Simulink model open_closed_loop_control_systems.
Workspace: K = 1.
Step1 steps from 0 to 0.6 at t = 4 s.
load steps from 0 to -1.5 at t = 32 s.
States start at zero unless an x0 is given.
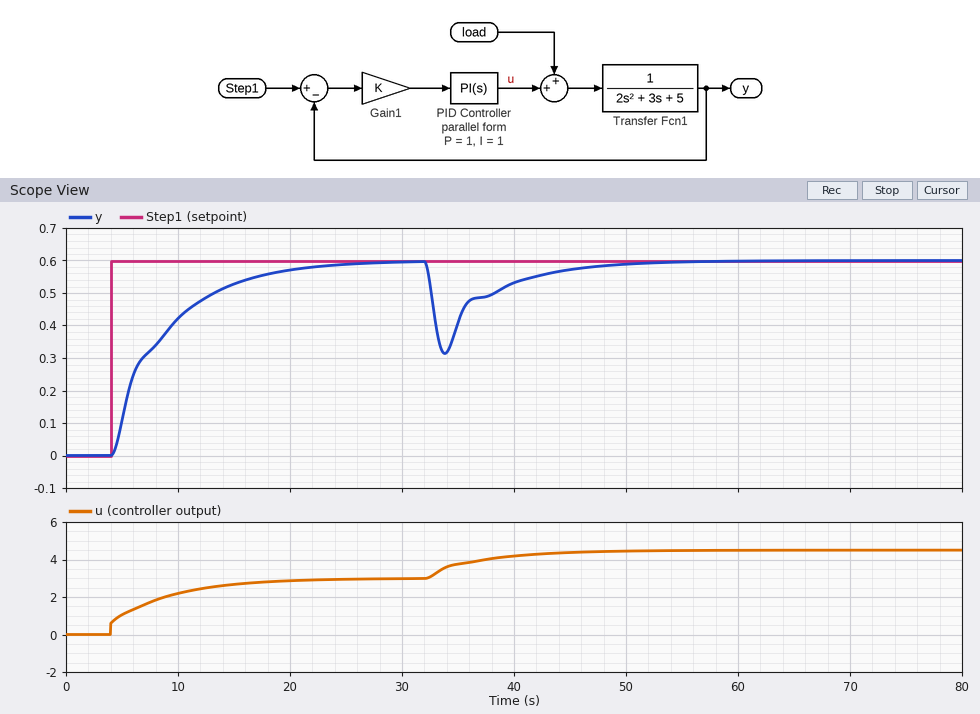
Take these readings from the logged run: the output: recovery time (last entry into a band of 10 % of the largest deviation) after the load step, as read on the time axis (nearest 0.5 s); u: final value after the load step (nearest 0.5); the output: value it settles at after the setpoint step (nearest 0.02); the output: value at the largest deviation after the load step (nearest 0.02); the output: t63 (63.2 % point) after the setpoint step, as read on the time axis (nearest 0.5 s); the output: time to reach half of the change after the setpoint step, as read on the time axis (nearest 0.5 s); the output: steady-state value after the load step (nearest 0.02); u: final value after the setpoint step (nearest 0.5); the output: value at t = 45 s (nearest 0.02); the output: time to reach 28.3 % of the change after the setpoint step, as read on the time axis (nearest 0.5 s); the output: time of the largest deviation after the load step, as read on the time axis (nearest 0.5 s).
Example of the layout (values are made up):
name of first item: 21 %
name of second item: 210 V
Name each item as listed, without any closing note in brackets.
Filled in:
the output: recovery time (last entry into a band of 10 % of the largest deviation) after the load step, as read on the time axis: 45.0 s
u: final value after the load step: 4.5
the output: value it settles at after the setpoint step: 0.60
the output: value at the largest deviation after the load step: 0.32
the output: t63 (63.2 % point) after the setpoint step, as read on the time axis: 9.0 s
the output: time to reach half of the change after the setpoint step, as read on the time axis: 7.0 s
the output: steady-state value after the load step: 0.60
u: final value after the setpoint step: 3.0
the output: value at t = 45 s: 0.58
the output: time to reach 28.3 % of the change after the setpoint step, as read on the time axis: 5.5 s
the output: time of the largest deviation after the load step, as read on the time axis: 34.0 s
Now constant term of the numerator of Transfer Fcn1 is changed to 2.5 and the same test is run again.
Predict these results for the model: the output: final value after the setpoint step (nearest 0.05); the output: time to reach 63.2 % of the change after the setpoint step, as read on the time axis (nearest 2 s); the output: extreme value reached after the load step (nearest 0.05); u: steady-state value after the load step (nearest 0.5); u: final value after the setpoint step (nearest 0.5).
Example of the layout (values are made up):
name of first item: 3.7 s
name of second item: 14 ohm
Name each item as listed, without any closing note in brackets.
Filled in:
the output: final value after the setpoint step: 0.60
the output: time to reach 63.2 % of the change after the setpoint step, as read on the time axis: 6 s
the output: extreme value reached after the load step: 0.05
u: steady-state value after the load step: 2.5
u: final value after the setpoint step: 1.0
